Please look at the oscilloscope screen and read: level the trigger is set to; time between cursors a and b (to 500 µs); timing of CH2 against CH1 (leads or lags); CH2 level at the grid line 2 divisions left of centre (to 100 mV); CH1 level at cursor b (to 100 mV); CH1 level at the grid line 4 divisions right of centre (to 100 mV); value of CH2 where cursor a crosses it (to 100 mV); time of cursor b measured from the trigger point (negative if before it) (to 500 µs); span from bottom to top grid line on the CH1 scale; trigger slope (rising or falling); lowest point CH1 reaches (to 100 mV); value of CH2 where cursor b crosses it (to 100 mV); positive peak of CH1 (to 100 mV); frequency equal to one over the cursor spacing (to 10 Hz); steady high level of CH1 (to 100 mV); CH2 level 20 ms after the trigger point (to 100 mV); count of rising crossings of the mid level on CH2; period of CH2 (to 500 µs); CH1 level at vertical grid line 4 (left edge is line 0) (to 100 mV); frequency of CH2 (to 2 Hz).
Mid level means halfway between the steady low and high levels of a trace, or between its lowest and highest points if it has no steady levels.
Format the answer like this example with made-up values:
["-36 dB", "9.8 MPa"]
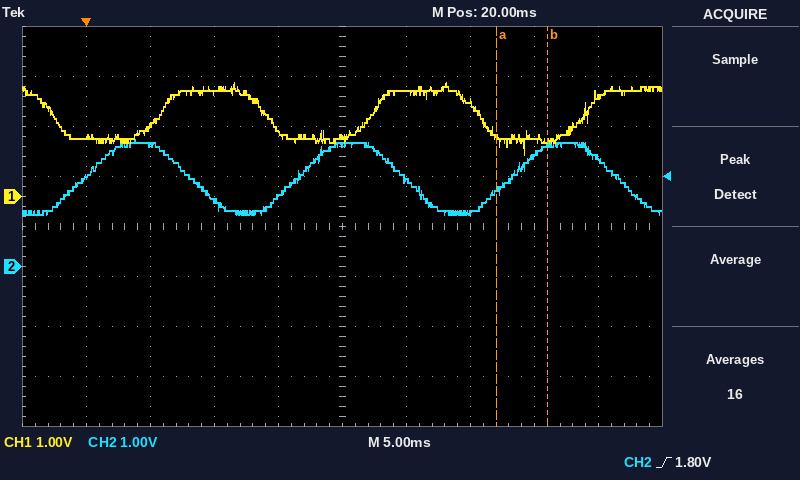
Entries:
["1.80 V", "4.0 ms", "leads", "1.3 V", "1.1 V", "2.0 V", "1.5 V", "+36.0 ms", "8 V", "rising", "800 mV", "2.4 V", "2.3 V", "250 Hz", "2.1 V", "2.4 V", "3", "16.5 ms", "1.3 V", "60 Hz"]
